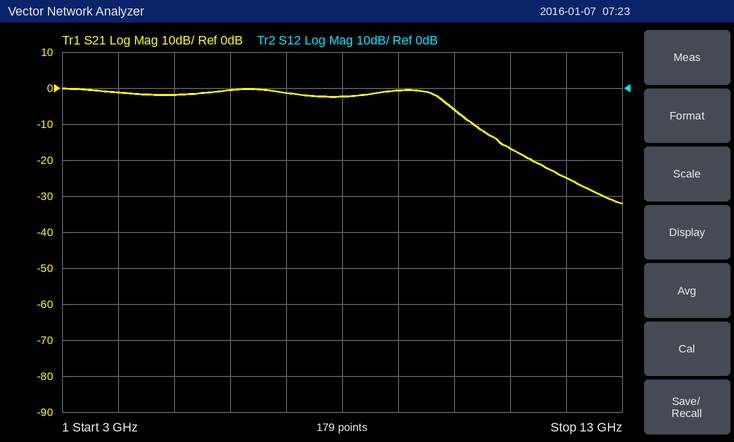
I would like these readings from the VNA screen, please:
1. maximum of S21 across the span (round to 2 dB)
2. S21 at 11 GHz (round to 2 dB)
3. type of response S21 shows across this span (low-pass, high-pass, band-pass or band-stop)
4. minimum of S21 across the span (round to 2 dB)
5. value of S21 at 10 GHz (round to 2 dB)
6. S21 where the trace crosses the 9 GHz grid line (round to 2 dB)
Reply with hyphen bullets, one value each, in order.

- 0 dB
- -16 dB
- low-pass
- -32 dB
- -6 dB
- 0 dB
